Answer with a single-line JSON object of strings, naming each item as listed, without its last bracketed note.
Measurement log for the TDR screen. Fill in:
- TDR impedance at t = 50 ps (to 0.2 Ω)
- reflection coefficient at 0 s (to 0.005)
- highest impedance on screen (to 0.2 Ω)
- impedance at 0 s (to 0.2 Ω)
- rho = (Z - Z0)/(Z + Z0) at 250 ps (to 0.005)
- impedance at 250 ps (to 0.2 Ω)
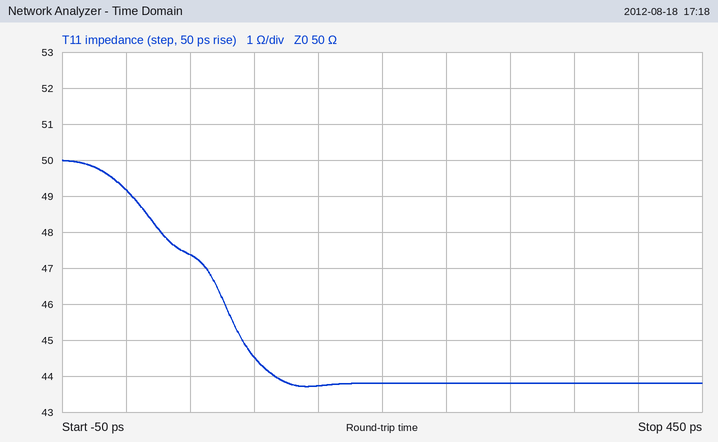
{"TDR impedance at t = 50 ps": "47.4 Ω", "reflection coefficient at 0 s": "-0.010", "highest impedance on screen": "50.0 Ω", "impedance at 0 s": "49.2 Ω", "rho = (Z - Z0)/(Z + Z0) at 250 ps": "-0.065", "impedance at 250 ps": "43.8 Ω"}
